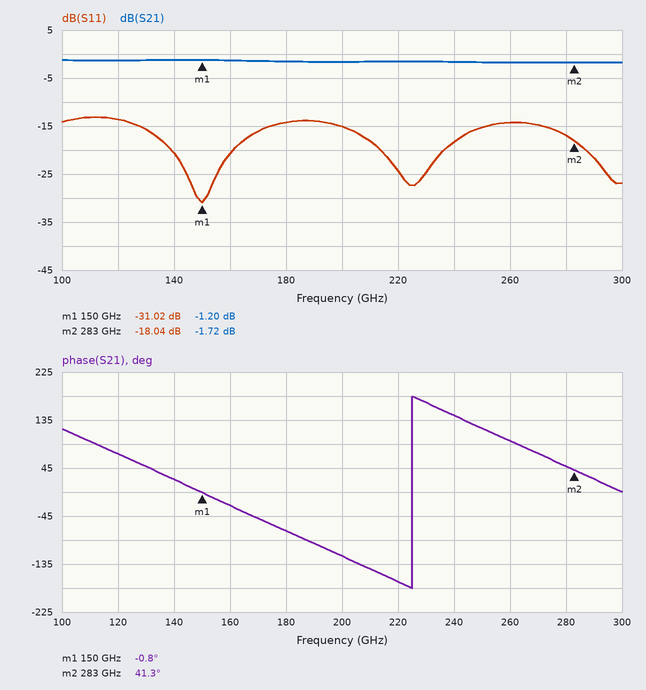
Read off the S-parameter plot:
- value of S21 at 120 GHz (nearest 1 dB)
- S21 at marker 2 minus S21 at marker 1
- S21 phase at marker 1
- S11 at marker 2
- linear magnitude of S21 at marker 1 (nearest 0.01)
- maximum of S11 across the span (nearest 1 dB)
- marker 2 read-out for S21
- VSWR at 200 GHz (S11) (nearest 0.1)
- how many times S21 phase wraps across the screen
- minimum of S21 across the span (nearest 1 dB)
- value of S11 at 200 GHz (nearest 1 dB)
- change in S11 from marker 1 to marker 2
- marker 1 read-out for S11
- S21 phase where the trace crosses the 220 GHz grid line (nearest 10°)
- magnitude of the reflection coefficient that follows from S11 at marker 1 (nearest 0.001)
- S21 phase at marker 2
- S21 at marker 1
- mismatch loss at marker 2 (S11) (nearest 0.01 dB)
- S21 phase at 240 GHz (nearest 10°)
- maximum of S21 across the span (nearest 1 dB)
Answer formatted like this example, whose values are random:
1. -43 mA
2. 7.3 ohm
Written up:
1. -1 dB
2. -0.52 dB
3. -0.8°
4. -18.04 dB
5. 0.87
6. -13 dB
7. -1.72 dB
8. 1.4
9. 1
10. -2 dB
11. -15 dB
12. 12.98 dB
13. -31.02 dB
14. -170°
15. 0.028
16. 41.3°
17. -1.20 dB
18. 0.07 dB
19. 140°
20. -1 dB
